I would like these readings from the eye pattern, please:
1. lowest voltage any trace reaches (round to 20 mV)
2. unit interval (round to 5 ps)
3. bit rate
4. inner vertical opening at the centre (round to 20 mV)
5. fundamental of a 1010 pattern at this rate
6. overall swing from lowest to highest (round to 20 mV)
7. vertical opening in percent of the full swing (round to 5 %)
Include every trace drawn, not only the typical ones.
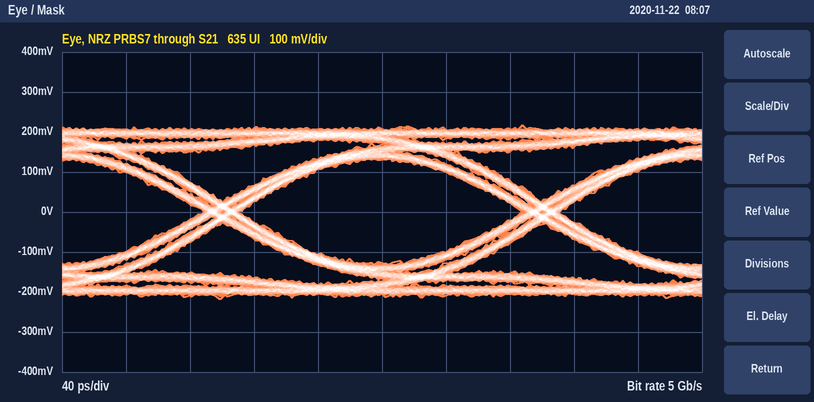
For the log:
-220 mV
200 ps
5 Gb/s
260 mV
2.5 GHz
440 mV
60 %
